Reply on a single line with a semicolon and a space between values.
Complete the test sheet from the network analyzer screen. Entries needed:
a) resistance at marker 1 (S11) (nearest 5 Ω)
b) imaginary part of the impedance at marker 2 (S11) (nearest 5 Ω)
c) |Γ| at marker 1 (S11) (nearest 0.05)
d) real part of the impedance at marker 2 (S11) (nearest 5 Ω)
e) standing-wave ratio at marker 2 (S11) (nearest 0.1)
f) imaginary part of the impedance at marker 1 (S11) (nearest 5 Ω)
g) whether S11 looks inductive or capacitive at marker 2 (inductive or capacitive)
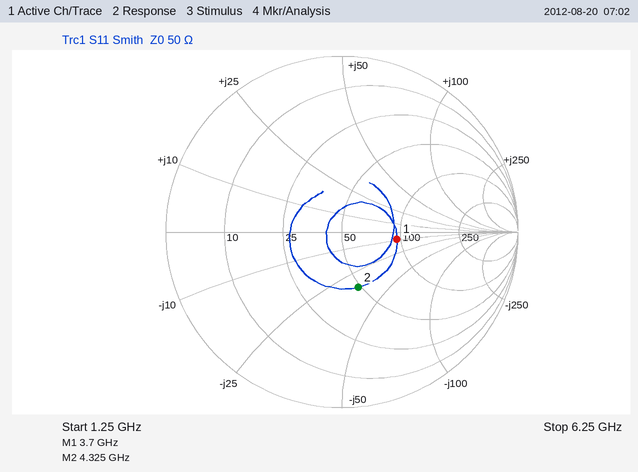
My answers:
95 Ω; -35 Ω; 0.30; 50 Ω; 2.0; -10 Ω; capacitive
